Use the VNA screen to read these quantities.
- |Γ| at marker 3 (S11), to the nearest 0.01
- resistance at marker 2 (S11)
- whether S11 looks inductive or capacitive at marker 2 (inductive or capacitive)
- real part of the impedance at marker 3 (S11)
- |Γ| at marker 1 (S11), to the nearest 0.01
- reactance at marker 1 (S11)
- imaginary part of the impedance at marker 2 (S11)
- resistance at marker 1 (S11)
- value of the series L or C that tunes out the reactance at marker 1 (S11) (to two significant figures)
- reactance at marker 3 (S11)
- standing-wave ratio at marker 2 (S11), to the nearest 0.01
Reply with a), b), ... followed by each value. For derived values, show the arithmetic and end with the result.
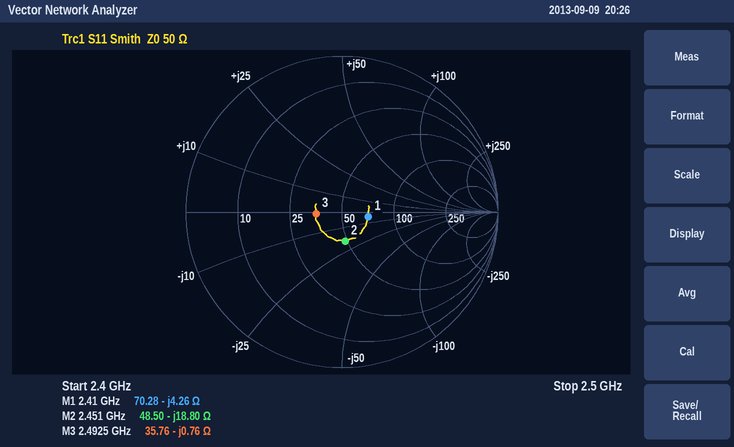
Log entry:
a) 0.17
b) 48.50 Ω
c) capacitive
d) 35.76 Ω
e) 0.17
f) -4.26 Ω
g) -18.80 Ω
h) 70.28 Ω
i) L = 4.26 Ω/(2π × 2.41 GHz) ≈ 281 pH, so 280 pH to two significant figures
j) -0.76 Ω
k) 1.46
